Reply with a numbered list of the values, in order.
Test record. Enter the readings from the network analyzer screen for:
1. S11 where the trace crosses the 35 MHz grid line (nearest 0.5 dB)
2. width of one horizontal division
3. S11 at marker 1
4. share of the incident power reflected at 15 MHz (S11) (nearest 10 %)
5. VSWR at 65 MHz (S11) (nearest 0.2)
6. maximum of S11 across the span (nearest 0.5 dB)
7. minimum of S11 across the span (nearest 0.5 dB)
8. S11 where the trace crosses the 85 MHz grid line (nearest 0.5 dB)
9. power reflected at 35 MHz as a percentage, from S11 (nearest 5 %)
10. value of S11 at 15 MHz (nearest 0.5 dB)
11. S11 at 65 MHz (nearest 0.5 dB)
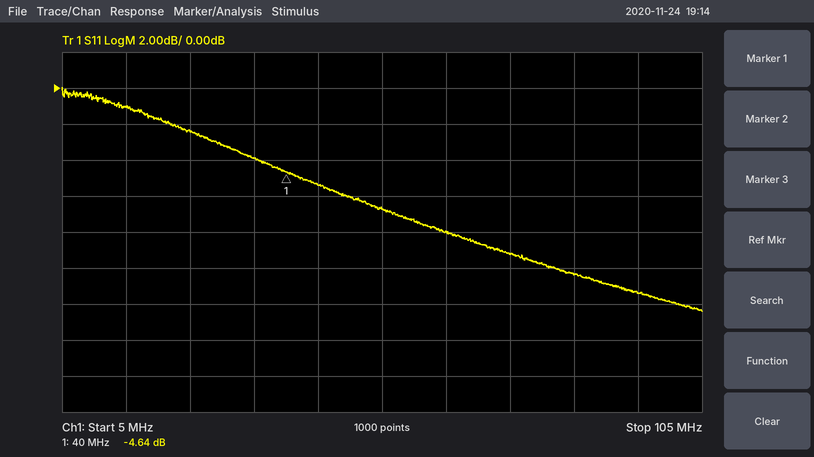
1. -4.0 dB
2. 10 MHz
3. -4.64 dB
4. 80 %
5. 2.4
6. 0.0 dB
7. -12.5 dB
8. -10.5 dB
9. 40 %
10. -1.0 dB
11. -8.0 dB
